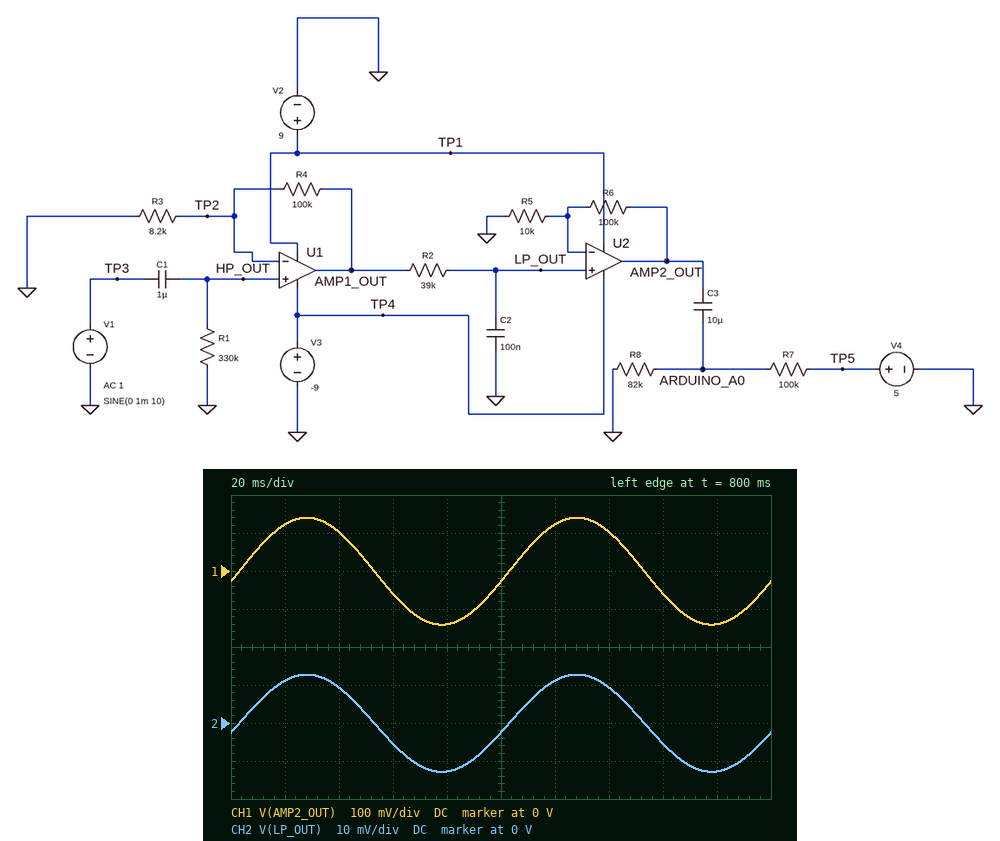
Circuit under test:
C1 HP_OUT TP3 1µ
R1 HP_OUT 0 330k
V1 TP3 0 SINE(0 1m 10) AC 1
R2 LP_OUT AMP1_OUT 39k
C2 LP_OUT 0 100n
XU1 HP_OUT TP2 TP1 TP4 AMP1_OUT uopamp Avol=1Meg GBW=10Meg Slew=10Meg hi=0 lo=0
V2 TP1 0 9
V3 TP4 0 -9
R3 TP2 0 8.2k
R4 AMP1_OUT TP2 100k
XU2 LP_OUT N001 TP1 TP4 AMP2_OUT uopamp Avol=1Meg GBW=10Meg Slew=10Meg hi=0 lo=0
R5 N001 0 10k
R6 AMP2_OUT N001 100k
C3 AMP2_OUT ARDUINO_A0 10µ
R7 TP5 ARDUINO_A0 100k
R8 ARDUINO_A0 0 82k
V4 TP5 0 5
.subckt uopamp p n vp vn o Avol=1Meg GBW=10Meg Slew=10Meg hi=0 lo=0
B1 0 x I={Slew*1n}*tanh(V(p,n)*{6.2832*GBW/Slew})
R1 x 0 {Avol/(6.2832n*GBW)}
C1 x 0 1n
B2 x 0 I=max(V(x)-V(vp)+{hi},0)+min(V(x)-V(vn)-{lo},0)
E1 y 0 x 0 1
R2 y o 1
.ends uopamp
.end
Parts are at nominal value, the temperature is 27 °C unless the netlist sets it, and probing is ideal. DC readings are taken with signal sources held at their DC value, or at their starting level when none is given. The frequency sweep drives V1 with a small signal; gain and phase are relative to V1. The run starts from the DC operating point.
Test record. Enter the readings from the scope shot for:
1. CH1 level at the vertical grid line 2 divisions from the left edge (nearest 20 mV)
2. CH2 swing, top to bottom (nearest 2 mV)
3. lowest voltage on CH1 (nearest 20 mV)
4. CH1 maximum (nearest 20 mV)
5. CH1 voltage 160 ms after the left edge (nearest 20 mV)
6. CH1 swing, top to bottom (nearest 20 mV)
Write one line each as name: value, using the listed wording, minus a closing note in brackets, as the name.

CH1 level at the vertical grid line 2 divisions from the left edge: 100 mV
CH2 swing, top to bottom: 26 mV
lowest voltage on CH1: -140 mV
CH1 maximum: 140 mV
CH1 voltage 160 ms after the left edge: -60 mV
CH1 swing, top to bottom: 280 mV
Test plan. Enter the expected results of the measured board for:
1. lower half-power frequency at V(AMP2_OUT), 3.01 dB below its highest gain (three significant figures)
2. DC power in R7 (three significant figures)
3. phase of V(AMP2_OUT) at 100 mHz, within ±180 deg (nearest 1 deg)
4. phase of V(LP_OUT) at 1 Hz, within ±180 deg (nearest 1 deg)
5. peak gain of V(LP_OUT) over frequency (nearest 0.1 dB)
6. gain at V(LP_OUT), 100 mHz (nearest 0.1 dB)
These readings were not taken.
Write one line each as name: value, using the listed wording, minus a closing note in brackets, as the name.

lower half-power frequency at V(AMP2_OUT), 3.01 dB below its highest gain: 471 mHz
DC power in R7: 75.5 µW
phase of V(AMP2_OUT) at 100 mHz, within ±180 deg: 78 deg
phase of V(LP_OUT) at 1 Hz, within ±180 deg: 24 deg
peak gain of V(LP_OUT) over frequency: 22.3 dB
gain at V(LP_OUT), 100 mHz: 8.6 dB
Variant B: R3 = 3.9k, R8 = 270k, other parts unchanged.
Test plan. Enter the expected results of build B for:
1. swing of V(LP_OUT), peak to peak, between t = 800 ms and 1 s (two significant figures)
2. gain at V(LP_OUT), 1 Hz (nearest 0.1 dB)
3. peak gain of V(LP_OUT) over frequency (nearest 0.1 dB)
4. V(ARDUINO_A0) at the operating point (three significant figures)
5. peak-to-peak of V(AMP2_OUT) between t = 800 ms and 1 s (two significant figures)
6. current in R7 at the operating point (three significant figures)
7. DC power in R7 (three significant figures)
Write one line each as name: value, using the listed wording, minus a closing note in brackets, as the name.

swing of V(LP_OUT), peak to peak, between t = 800 ms and 1 s: 52 mV
gain at V(LP_OUT), 1 Hz: 27.6 dB
peak gain of V(LP_OUT) over frequency: 28.4 dB
V(ARDUINO_A0) at the operating point: 3.65 V
peak-to-peak of V(AMP2_OUT) between t = 800 ms and 1 s: 570 mV
current in R7 at the operating point: 13.5 µA
DC power in R7: 18.3 µW
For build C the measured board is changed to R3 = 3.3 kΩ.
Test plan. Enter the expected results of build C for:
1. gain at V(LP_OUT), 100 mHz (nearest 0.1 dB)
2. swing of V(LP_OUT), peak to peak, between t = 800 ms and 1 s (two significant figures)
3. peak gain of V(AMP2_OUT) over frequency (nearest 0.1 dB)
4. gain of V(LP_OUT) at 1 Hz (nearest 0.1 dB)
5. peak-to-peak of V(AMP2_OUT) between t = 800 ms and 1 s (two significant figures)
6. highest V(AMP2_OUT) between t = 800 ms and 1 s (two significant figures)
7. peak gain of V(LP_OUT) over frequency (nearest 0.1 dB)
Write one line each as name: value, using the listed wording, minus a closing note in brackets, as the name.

gain at V(LP_OUT), 100 mHz: 16.1 dB
swing of V(LP_OUT), peak to peak, between t = 800 ms and 1 s: 61 mV
peak gain of V(AMP2_OUT) over frequency: 50.6 dB
gain of V(LP_OUT) at 1 Hz: 29.0 dB
peak-to-peak of V(AMP2_OUT) between t = 800 ms and 1 s: 670 mV
highest V(AMP2_OUT) between t = 800 ms and 1 s: 330 mV
peak gain of V(LP_OUT) over frequency: 29.8 dB
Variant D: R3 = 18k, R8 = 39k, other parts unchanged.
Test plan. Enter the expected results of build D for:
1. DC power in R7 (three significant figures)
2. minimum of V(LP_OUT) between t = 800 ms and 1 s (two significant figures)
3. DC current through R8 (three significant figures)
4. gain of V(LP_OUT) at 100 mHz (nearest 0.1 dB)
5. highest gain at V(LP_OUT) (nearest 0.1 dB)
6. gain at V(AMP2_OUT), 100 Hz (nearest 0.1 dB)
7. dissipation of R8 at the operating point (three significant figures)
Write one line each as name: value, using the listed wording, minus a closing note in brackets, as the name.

DC power in R7: 129 µW
minimum of V(LP_OUT) between t = 800 ms and 1 s: -6.4 mV
DC current through R8: 36.0 µA
gain of V(LP_OUT) at 100 mHz: 2.5 dB
highest gain at V(LP_OUT): 16.2 dB
gain at V(AMP2_OUT), 100 Hz: 28.7 dB
dissipation of R8 at the operating point: 50.5 µW
